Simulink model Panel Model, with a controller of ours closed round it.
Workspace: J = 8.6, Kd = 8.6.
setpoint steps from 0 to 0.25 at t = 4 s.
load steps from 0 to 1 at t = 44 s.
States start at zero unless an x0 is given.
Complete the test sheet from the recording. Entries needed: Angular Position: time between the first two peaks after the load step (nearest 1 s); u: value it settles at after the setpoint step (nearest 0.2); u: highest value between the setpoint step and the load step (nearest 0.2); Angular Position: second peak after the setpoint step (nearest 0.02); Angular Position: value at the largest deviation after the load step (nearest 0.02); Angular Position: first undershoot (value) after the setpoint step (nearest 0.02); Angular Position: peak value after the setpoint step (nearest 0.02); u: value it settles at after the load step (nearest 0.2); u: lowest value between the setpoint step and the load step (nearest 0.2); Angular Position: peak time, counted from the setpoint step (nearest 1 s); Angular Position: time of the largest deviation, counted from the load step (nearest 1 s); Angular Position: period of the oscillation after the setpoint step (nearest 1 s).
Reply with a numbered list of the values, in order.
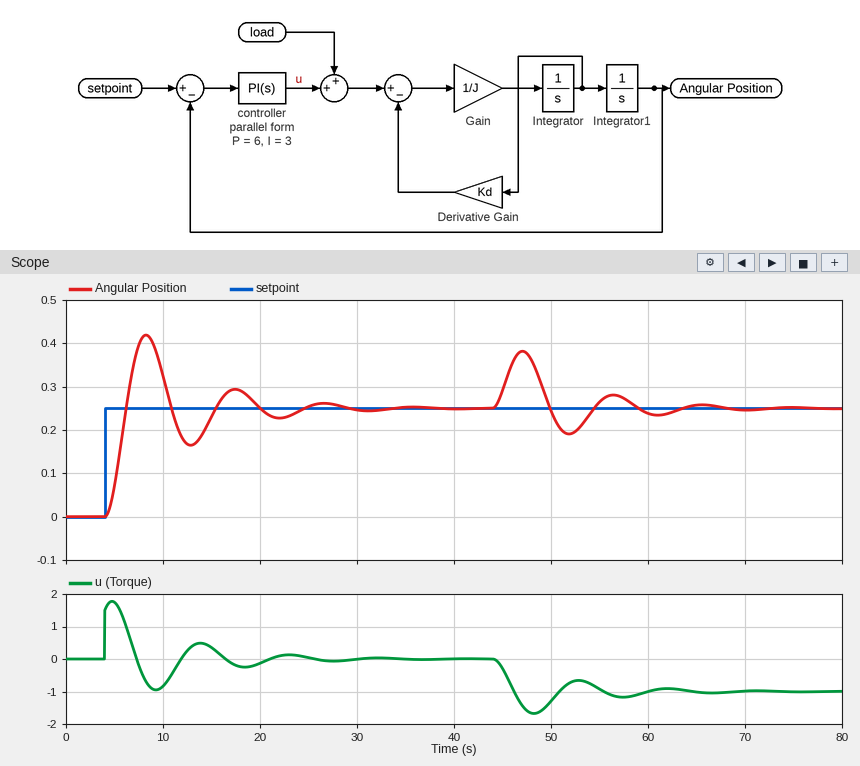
1. 9 s
2. 0.0
3. 1.8
4. 0.30
5. 0.38
6. 0.16
7. 0.42
8. -1.0
9. -1.0
10. 4 s
11. 3 s
12. 9 s
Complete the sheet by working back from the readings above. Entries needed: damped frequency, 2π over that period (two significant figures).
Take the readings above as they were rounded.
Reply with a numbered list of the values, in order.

1. 0.70 rad/s
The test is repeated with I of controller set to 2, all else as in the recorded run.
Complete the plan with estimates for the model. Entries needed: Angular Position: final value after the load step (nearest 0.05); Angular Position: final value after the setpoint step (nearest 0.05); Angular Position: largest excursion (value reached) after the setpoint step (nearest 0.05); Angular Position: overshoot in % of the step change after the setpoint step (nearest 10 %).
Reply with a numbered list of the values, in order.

1. 0.25
2. 0.25
3. 0.40
4. 50 %
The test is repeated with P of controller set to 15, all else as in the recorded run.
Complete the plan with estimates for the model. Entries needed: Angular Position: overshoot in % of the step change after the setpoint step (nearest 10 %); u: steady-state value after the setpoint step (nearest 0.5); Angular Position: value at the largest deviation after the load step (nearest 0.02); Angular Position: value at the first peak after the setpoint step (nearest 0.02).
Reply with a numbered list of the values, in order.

1. 50 %
2. 0.0
3. 0.32
4. 0.36
